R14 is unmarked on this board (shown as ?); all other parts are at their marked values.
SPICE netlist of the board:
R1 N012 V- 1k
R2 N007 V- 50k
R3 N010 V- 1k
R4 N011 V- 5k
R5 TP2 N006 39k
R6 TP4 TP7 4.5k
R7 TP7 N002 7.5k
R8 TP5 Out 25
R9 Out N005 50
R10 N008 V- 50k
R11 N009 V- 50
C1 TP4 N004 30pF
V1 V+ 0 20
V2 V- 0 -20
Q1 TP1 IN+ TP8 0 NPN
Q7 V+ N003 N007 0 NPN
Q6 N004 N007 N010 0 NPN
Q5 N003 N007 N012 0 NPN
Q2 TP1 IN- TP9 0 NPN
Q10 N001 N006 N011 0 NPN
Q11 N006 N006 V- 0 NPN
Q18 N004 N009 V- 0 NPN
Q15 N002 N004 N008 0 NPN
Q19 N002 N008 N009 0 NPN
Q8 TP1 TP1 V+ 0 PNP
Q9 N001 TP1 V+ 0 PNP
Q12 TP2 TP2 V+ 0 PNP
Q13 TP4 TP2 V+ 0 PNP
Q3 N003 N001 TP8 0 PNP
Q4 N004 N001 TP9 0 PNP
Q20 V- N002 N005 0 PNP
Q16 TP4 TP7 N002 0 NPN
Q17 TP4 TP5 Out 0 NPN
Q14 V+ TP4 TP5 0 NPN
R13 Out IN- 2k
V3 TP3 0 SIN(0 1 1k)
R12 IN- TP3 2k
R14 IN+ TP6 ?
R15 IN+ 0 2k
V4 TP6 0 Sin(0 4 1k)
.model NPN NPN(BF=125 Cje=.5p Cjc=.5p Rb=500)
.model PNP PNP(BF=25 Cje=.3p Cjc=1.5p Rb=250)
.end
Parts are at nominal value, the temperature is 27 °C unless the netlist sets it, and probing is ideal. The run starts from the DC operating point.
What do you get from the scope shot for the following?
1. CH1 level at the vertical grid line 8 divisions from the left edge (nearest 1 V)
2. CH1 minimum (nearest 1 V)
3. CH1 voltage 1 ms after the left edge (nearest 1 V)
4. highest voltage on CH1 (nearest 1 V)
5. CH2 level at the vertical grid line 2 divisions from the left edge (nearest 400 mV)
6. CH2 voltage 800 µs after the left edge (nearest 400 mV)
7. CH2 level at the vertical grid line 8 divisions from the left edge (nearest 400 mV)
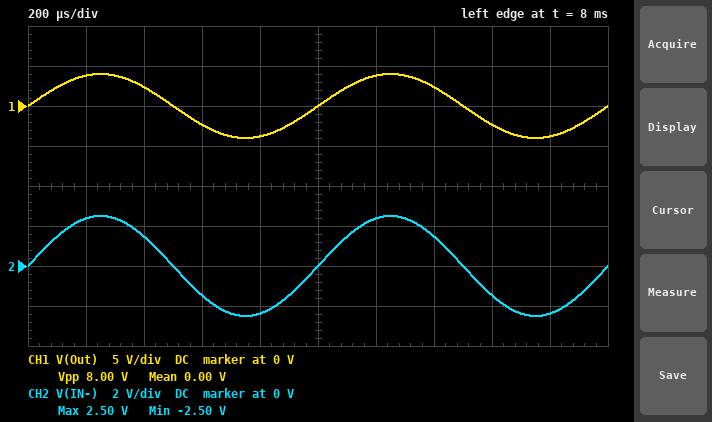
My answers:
-2 V
-4 V
0 V
4 V
1.6 V
-2.4 V
-1.6 V
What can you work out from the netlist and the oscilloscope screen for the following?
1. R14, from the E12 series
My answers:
1.2 kΩ
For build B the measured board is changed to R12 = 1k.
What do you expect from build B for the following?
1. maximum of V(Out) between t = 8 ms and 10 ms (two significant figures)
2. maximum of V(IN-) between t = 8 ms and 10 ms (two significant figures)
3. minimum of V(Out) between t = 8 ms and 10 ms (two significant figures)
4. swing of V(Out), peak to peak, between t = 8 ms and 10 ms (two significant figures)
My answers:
5.5 V
2.5 V
-5.5 V
11 V
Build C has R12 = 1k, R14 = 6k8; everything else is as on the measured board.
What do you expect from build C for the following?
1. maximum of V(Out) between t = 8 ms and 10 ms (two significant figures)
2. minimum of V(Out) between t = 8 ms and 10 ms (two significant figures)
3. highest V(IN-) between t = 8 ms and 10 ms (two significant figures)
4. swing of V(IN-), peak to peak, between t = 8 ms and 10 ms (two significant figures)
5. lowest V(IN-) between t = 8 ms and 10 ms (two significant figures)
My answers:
730 mV
-730 mV
910 mV
1.8 V
-910 mV
